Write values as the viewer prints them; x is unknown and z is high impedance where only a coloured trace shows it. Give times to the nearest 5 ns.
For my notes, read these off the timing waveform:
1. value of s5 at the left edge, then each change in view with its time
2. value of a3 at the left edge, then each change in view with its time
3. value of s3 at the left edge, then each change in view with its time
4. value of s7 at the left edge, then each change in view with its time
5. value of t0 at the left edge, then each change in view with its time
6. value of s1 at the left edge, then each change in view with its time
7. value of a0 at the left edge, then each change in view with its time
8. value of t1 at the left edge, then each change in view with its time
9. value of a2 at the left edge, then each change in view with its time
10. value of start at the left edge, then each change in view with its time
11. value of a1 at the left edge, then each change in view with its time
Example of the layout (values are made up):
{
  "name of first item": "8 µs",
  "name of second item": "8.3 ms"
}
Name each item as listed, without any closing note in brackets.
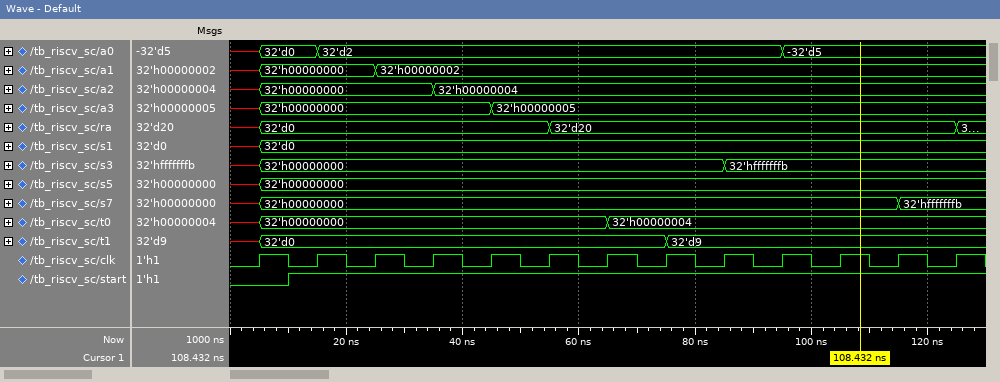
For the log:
{
  "value of s5 at the left edge, then each change in view with its time": "x, 32'h00000000 at 5 ns",
  "value of a3 at the left edge, then each change in view with its time": "x, 32'h00000000 at 5 ns, 32'h00000005 at 45 ns",
  "value of s3 at the left edge, then each change in view with its time": "x, 32'h00000000 at 5 ns, 32'hfffffffb at 85 ns",
  "value of s7 at the left edge, then each change in view with its time": "x, 32'h00000000 at 5 ns, 32'hfffffffb at 115 ns",
  "value of t0 at the left edge, then each change in view with its time": "x, 32'h00000000 at 5 ns, 32'h00000004 at 65 ns",
  "value of s1 at the left edge, then each change in view with its time": "x, 32'd0 at 5 ns",
  "value of a0 at the left edge, then each change in view with its time": "x, 32'd0 at 5 ns, 32'd2 at 15 ns, -32'd5 at 95 ns",
  "value of t1 at the left edge, then each change in view with its time": "x, 32'd0 at 5 ns, 32'd9 at 75 ns",
  "value of a2 at the left edge, then each change in view with its time": "x, 32'h00000000 at 5 ns, 32'h00000004 at 35 ns",
  "value of start at the left edge, then each change in view with its time": "0, 1 at 10 ns",
  "value of a1 at the left edge, then each change in view with its time": "x, 32'h00000000 at 5 ns, 32'h00000002 at 25 ns"
}
